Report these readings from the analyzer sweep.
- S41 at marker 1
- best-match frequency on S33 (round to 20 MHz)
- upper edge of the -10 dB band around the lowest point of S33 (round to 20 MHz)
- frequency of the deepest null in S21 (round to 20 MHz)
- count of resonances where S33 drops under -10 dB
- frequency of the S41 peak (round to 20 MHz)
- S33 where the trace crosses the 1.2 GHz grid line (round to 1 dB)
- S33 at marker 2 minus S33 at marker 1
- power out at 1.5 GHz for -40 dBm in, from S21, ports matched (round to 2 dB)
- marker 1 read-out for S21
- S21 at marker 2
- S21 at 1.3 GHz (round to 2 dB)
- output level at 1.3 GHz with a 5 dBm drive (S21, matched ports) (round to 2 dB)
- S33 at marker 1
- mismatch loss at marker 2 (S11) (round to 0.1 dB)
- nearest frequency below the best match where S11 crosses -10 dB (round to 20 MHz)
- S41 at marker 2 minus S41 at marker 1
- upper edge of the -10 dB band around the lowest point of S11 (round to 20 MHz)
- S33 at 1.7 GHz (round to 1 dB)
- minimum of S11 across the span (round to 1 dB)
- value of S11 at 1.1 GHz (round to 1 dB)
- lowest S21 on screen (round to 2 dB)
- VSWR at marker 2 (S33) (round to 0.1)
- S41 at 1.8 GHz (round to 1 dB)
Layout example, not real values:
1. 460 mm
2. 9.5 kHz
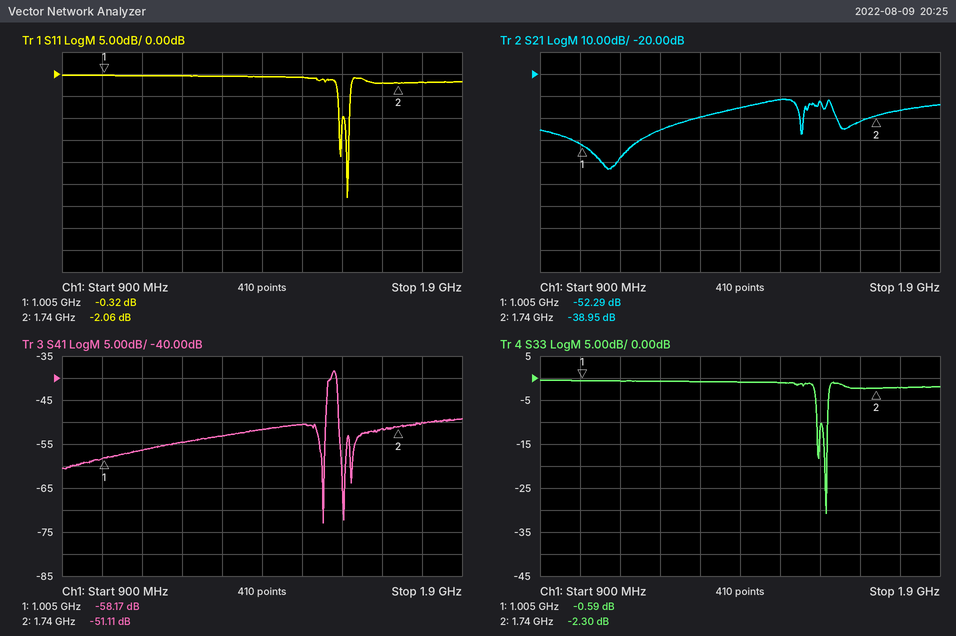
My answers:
1. -58.17 dB
2. 1.62 GHz
3. 1.62 GHz
4. 1.08 GHz
5. 2
6. 1.58 GHz
7. -1 dB
8. -1.71 dB
9. -72 dBm
10. -52.29 dB
11. -38.95 dB
12. -40 dB
13. -34 dBm
14. -0.59 dB
15. 4.2 dB
16. 1.60 GHz
17. 7.06 dB
18. 1.62 GHz
19. -2 dB
20. -28 dB
21. 0 dB
22. -64 dB
23. 7.6
24. -50 dB
